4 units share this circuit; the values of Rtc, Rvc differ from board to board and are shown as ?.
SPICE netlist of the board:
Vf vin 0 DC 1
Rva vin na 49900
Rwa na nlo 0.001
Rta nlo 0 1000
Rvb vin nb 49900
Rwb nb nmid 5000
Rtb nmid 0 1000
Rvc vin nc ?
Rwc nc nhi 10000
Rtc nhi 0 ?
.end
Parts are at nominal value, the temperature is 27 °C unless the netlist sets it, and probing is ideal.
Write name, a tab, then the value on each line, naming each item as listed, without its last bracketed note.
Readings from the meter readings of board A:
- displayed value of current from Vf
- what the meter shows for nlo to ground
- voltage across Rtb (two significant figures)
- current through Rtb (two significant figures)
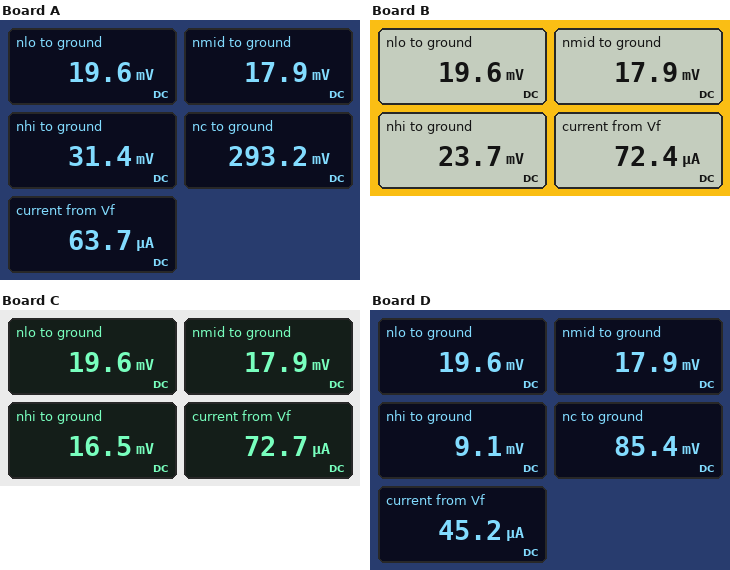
displayed value of current from Vf	63.7 µA
what the meter shows for nlo to ground	19.6 mV
voltage across Rtb	18 mV
current through Rtb	18 µA
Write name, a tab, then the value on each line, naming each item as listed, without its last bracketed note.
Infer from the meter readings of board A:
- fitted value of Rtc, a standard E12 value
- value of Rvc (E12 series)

fitted value of Rtc, a standard E12 value	1.2 kΩ
value of Rvc	27 kΩ
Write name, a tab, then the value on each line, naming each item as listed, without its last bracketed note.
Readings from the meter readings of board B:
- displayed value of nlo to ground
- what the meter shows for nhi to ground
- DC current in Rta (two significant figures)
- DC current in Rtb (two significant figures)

displayed value of nlo to ground	19.6 mV
what the meter shows for nhi to ground	23.7 mV
DC current in Rta	20 µA
DC current in Rtb	18 µA
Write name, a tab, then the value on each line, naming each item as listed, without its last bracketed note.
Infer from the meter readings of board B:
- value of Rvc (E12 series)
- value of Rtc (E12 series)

value of Rvc	18 kΩ
value of Rtc	680 Ω
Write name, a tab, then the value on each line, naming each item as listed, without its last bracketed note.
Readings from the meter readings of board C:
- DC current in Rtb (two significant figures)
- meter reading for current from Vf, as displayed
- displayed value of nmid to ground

DC current in Rtb	18 µA
meter reading for current from Vf, as displayed	72.7 µA
displayed value of nmid to ground	17.9 mV
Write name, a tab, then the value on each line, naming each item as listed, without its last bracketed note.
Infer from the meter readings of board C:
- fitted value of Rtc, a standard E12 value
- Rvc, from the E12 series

fitted value of Rtc, a standard E12 value	470 Ω
Rvc, from the E12 series	18 kΩ
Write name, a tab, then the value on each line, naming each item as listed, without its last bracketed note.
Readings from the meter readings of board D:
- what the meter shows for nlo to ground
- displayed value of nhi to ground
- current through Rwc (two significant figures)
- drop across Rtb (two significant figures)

what the meter shows for nlo to ground	19.6 mV
displayed value of nhi to ground	9.1 mV
current through Rwc	7.6 µA
drop across Rtb	18 mV
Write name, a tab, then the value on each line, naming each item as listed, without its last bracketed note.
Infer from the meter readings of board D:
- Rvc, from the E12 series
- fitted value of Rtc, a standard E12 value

Rvc, from the E12 series	120 kΩ
fitted value of Rtc, a standard E12 value	1.2 kΩ
